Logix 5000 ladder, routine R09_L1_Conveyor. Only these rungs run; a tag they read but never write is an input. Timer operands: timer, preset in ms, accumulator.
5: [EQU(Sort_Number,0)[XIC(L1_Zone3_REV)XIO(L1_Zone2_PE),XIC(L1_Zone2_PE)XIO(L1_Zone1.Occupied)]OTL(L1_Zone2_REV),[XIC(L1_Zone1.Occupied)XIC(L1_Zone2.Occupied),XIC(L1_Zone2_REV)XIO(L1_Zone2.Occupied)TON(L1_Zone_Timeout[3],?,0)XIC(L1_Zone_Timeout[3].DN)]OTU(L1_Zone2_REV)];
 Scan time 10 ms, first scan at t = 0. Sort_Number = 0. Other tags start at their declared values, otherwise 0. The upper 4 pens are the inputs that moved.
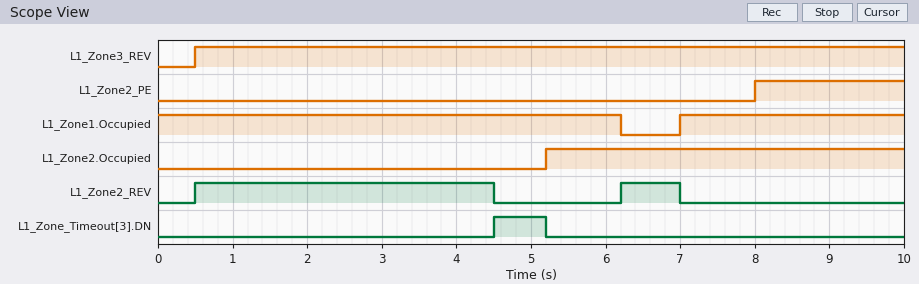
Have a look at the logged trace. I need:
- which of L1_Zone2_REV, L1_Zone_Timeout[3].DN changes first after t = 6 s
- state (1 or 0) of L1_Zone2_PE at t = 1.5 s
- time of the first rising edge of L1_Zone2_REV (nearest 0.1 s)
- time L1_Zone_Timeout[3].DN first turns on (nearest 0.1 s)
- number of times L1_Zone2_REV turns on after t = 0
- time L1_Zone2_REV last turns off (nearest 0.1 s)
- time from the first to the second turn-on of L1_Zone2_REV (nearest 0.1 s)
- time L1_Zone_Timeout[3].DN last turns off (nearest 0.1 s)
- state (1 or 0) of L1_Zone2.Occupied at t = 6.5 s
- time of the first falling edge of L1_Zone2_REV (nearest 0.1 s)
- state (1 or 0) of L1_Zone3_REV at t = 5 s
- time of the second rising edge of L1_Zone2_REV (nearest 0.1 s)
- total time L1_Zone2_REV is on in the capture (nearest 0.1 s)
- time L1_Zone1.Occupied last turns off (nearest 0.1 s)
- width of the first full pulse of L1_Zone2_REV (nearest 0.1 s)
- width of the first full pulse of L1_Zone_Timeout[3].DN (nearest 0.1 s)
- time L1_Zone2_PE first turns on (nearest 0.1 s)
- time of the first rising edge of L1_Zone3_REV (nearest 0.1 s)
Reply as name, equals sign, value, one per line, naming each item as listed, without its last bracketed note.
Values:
which of L1_Zone2_REV, L1_Zone_Timeout[3].DN changes first after t = 6 s = L1_Zone2_REV
state (1 or 0) of L1_Zone2_PE at t = 1.5 s = 0
time of the first rising edge of L1_Zone2_REV = 0.5 s
time L1_Zone_Timeout[3].DN first turns on = 4.5 s
number of times L1_Zone2_REV turns on after t = 0 = 2
time L1_Zone2_REV last turns off = 7.0 s
time from the first to the second turn-on of L1_Zone2_REV = 5.7 s
time L1_Zone_Timeout[3].DN last turns off = 5.2 s
state (1 or 0) of L1_Zone2.Occupied at t = 6.5 s = 1
time of the first falling edge of L1_Zone2_REV = 4.5 s
state (1 or 0) of L1_Zone3_REV at t = 5 s = 1
time of the second rising edge of L1_Zone2_REV = 6.2 s
total time L1_Zone2_REV is on in the capture = 4.8 s
time L1_Zone1.Occupied last turns off = 6.2 s
width of the first full pulse of L1_Zone2_REV = 4.0 s
width of the first full pulse of L1_Zone_Timeout[3].DN = 0.7 s
time L1_Zone2_PE first turns on = 8.0 s
time of the first rising edge of L1_Zone3_REV = 0.5 s
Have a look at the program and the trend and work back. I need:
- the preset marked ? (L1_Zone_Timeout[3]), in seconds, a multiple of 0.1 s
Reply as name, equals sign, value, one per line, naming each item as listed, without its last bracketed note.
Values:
the preset marked ? (L1_Zone_Timeout[3]), in seconds, a multiple of 0.1 s = 4.0 s
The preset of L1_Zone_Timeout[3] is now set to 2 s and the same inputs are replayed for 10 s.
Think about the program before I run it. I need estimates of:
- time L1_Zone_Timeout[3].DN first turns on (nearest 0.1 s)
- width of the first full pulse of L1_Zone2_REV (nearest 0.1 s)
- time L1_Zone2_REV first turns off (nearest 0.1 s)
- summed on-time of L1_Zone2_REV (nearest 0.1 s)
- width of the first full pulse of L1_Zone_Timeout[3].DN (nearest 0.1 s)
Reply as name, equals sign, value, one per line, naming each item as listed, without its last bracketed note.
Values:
time L1_Zone_Timeout[3].DN first turns on = 2.5 s
width of the first full pulse of L1_Zone2_REV = 2.0 s
time L1_Zone2_REV first turns off = 2.5 s
summed on-time of L1_Zone2_REV = 2.8 s
width of the first full pulse of L1_Zone_Timeout[3].DN = 2.7 s
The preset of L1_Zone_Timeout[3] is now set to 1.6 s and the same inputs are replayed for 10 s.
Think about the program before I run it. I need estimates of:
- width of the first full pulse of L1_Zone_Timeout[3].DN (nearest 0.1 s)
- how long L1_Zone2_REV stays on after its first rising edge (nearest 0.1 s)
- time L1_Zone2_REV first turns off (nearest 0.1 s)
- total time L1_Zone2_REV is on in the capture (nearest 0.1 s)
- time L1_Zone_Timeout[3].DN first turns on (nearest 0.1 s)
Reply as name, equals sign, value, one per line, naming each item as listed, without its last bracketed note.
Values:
width of the first full pulse of L1_Zone_Timeout[3].DN = 3.1 s
how long L1_Zone2_REV stays on after its first rising edge = 1.6 s
time L1_Zone2_REV first turns off = 2.1 s
total time L1_Zone2_REV is on in the capture = 2.4 s
time L1_Zone_Timeout[3].DN first turns on = 2.1 s
